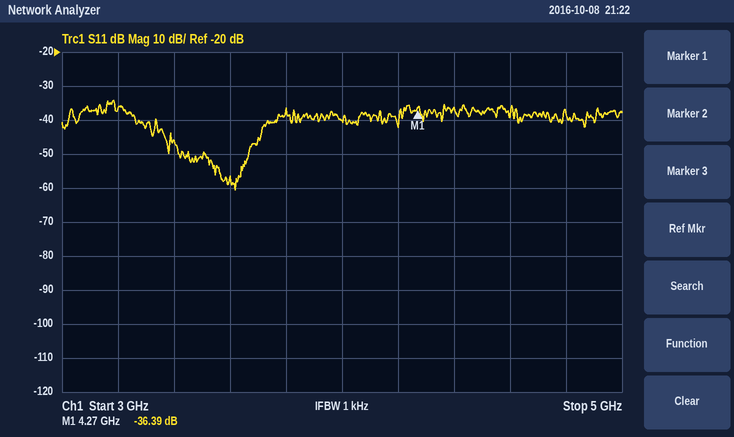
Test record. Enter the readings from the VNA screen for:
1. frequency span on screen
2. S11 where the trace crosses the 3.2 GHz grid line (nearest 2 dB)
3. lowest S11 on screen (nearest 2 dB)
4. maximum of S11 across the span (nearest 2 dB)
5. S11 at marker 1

2 GHz
-36 dB
-60 dB
-34 dB
-36.39 dB
